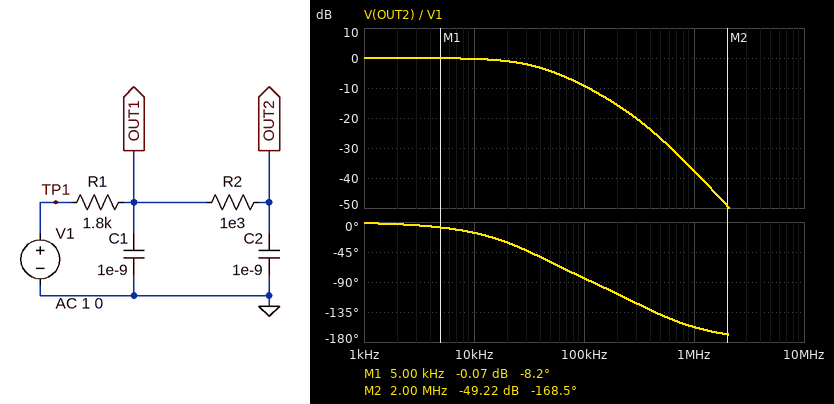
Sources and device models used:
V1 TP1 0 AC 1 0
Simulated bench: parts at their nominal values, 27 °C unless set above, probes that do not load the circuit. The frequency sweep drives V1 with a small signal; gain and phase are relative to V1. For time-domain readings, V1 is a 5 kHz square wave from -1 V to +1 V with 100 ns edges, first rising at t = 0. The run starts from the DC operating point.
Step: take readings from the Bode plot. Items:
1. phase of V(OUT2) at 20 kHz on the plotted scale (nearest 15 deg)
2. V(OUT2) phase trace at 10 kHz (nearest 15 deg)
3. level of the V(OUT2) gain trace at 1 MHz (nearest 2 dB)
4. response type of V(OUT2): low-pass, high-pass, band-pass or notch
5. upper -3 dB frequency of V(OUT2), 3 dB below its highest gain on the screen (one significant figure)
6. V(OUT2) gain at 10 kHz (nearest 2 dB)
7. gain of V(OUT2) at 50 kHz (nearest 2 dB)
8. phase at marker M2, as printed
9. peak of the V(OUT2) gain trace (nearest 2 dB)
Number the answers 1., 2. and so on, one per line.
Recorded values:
1. -30 deg
2. -15 deg
3. -38 dB
4. low-pass
5. 40 kHz
6. 0 dB
7. -4 dB
8. -168.5 deg
9. 0 dB
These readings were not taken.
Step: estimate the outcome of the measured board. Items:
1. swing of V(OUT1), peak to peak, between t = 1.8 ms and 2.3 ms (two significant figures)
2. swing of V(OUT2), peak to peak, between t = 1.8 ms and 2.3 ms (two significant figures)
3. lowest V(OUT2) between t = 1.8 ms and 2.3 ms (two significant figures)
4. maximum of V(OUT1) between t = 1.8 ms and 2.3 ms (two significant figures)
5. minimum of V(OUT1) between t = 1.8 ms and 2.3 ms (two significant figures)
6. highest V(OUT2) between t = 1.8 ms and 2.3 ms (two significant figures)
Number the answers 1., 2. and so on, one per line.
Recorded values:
1. 2.0 V
2. 2.0 V
3. -1.0 V
4. 1.0 V
5. -1.0 V
6. 1.0 V
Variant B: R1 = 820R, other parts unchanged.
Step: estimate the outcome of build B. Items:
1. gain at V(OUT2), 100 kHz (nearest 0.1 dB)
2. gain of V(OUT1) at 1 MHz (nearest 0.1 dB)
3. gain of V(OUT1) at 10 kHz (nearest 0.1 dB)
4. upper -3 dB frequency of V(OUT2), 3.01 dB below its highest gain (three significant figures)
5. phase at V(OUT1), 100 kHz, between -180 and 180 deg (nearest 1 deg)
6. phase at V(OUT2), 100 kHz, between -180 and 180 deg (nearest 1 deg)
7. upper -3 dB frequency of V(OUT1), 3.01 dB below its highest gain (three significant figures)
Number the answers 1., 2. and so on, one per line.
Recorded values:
1. -5.1 dB
2. -14.9 dB
3. -0.1 dB
4. 68.2 kHz
5. -36 deg
6. -68 deg
7. 84.8 kHz
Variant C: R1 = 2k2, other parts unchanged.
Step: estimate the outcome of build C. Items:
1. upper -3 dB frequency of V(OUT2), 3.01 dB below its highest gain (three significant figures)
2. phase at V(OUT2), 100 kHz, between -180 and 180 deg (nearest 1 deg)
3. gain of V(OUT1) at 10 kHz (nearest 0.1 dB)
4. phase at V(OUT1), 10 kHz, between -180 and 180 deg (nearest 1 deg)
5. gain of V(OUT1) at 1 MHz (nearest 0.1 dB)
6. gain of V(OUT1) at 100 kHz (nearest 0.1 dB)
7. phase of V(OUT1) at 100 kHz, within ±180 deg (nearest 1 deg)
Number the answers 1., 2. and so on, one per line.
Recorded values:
1. 31.9 kHz
2. -88 deg
3. -0.4 dB
4. -15 deg
5. -23.2 dB
6. -9.2 dB
7. -56 deg
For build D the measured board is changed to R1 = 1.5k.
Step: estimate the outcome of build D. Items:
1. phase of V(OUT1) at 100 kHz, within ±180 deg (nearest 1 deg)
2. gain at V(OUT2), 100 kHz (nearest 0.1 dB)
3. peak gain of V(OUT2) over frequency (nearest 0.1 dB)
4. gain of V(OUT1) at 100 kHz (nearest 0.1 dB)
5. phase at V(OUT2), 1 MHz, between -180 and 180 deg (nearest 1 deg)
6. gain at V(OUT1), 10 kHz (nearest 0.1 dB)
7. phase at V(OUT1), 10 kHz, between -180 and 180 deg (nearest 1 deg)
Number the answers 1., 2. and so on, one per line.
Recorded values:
1. -49 deg
2. -8.1 dB
3. 0 dB
4. -6.7 dB
5. -157 deg
6. -0.2 dB
7. -11 deg
